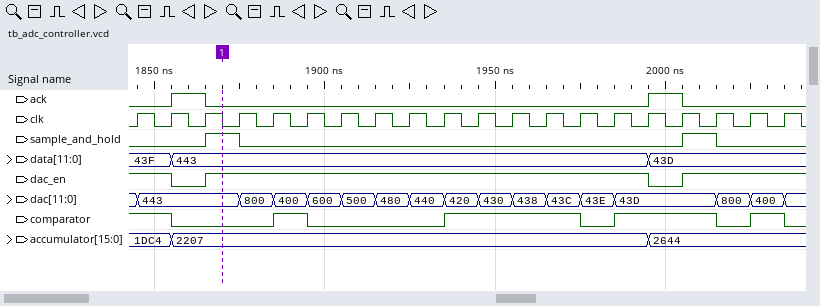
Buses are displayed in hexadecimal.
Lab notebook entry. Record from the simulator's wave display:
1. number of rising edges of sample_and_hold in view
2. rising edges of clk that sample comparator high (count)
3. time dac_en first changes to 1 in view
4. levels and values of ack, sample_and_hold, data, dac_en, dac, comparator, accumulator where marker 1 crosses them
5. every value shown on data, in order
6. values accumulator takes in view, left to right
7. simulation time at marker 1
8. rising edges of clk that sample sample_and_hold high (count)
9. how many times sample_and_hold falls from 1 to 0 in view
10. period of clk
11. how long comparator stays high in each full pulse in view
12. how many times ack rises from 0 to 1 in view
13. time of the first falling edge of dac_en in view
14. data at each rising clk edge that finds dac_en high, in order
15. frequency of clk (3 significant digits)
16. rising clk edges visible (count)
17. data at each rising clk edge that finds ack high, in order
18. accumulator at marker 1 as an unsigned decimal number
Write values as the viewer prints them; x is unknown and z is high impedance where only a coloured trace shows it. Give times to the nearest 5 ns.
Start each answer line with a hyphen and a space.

- 2
- 11
- 1865 ns
- ack=0, sample_and_hold=1, data=443, dac_en=1, dac=443, comparator=0, accumulator=2207
- 43F, 443, 43D
- 1DC4, 2207, 2644
- 1870 ns
- 2
- 2
- 10 ns
- 10 ns, 40 ns, 30 ns, 10 ns
- 2
- 1855 ns
- 43F, 43F, 443, 443, 443, 443, 443, 443, 443, 443, 443, 443, 443, 443, 443, 43D, 43D, 43D
- 100 MHz
- 20
- 443, 43D
- 8711
